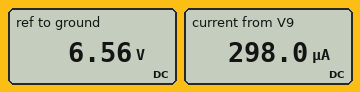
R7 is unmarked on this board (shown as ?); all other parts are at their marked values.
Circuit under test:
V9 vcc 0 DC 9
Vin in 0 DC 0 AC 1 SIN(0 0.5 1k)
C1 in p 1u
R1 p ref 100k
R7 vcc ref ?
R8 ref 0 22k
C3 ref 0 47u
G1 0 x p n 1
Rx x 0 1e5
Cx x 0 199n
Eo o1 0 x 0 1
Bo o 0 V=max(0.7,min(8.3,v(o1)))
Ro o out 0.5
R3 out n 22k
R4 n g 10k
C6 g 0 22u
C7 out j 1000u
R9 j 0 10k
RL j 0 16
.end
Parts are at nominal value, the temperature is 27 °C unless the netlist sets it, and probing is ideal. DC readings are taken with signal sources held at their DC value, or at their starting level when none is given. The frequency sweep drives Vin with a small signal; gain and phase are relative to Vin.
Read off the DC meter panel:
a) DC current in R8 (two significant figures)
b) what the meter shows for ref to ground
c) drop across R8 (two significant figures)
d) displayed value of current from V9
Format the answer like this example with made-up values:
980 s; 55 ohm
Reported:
300 µA; 6.56 V; 6.6 V; 298.0 µA
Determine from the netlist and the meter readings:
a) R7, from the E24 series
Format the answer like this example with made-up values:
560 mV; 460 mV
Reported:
8.2 kΩ
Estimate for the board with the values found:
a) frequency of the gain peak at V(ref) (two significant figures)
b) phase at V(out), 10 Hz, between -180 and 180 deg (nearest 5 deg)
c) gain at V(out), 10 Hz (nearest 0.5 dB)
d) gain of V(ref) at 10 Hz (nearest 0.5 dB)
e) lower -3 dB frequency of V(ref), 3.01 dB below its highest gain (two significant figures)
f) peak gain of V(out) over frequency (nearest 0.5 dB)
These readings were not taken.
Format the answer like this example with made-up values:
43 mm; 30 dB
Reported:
950 mHz; 10 deg; 10.0 dB; -49.5 dB; 350 mHz; 10.0 dB
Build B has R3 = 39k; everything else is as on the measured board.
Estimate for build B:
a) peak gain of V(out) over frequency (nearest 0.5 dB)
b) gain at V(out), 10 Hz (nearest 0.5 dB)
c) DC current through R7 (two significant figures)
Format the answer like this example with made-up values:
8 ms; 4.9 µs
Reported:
14.0 dB; 13.5 dB; 300 µA
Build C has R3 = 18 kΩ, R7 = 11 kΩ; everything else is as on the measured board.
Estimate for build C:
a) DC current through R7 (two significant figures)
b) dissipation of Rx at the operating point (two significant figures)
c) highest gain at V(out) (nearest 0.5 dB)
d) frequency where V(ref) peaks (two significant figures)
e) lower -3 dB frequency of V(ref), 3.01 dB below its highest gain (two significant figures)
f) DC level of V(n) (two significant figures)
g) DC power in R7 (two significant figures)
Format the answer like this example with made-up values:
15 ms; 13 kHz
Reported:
270 µA; 360 µW; 9.0 dB; 860 mHz; 310 mHz; 6.0 V; 820 µW
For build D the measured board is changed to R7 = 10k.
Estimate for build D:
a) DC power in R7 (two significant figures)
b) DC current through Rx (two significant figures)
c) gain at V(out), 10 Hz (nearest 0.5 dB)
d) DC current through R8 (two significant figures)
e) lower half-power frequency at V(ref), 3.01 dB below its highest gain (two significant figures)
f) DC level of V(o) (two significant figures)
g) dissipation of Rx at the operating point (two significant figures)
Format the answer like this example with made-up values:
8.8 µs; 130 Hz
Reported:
790 µW; 62 µA; 10.0 dB; 280 µA; 320 mHz; 6.2 V; 380 µW
